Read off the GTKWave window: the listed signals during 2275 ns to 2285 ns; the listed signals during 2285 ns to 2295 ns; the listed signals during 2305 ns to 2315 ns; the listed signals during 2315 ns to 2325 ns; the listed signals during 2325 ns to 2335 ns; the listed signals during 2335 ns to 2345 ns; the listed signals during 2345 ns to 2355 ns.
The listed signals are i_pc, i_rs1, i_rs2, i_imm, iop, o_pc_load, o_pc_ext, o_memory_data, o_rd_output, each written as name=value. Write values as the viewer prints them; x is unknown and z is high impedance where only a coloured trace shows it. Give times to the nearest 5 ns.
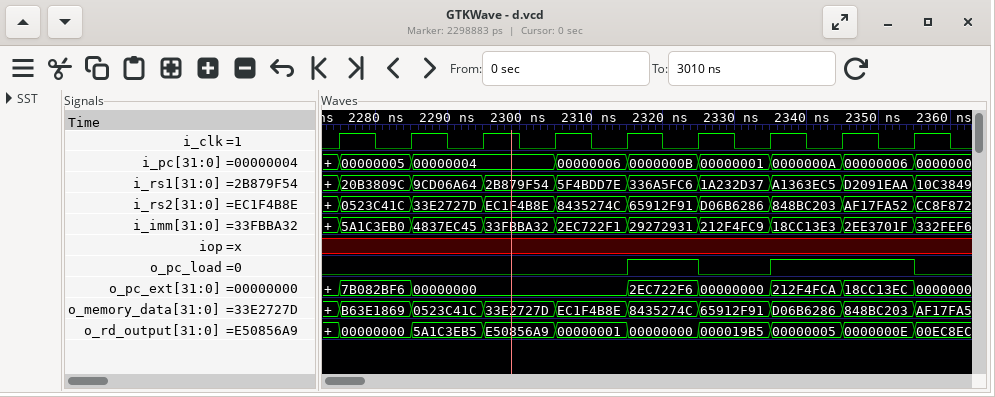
i_pc=00000005, i_rs1=20B3809C, i_rs2=0523C41C, i_imm=5A1C3EB0, iop=x, o_pc_load=0, o_pc_ext=7B082BF6, o_memory_data=B63E1869, o_rd_output=00000000
i_pc=00000004, i_rs1=9CD06A64, i_rs2=33E2727D, i_imm=4837EC45, iop=x, o_pc_load=0, o_pc_ext=00000000, o_memory_data=0523C41C, o_rd_output=5A1C3EB5
i_pc=00000006, i_rs1=5F4BDD7E, i_rs2=8435274C, i_imm=2EC722F1, iop=x, o_pc_load=0, o_pc_ext=00000000, o_memory_data=EC1F4B8E, o_rd_output=00000001
i_pc=0000000B, i_rs1=336A5FC6, i_rs2=65912F91, i_imm=29272931, iop=x, o_pc_load=1, o_pc_ext=2EC722F6, o_memory_data=8435274C, o_rd_output=00000000
i_pc=00000001, i_rs1=1A232D37, i_rs2=D06B6286, i_imm=212F4FC9, iop=x, o_pc_load=0, o_pc_ext=00000000, o_memory_data=65912F91, o_rd_output=000019B5
i_pc=0000000A, i_rs1=A1363EC5, i_rs2=848BC203, i_imm=18CC13E3, iop=x, o_pc_load=1, o_pc_ext=212F4FCA, o_memory_data=D06B6286, o_rd_output=00000005
i_pc=00000006, i_rs1=D2091EAA, i_rs2=AF17FA52, i_imm=2EE3701F, iop=x, o_pc_load=1, o_pc_ext=18CC13EC, o_memory_data=848BC203, o_rd_output=0000000E
